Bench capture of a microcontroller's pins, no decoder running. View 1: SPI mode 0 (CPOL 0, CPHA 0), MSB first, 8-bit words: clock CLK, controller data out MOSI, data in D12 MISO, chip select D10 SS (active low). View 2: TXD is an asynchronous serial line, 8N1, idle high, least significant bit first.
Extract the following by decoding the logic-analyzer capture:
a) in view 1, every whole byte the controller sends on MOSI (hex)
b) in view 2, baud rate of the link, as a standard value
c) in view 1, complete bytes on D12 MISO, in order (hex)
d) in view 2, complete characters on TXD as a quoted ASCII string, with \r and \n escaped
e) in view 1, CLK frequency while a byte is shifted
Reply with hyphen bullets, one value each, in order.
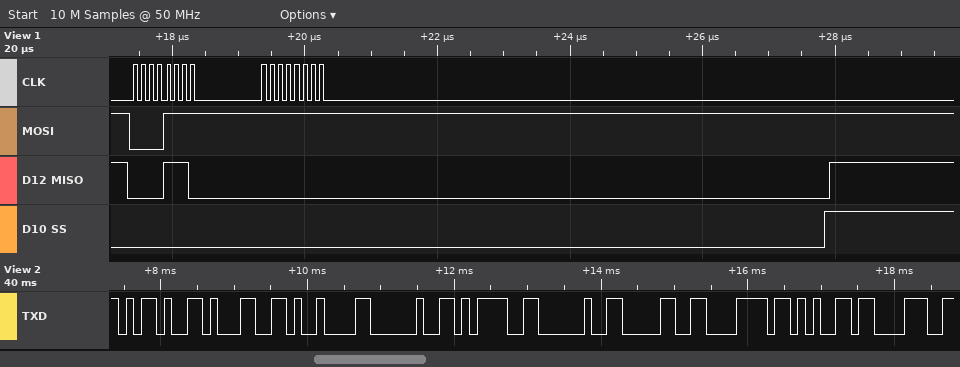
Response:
- 0F FF
- 9600 baud
- 0E 00
- "-1\t = 0xe8"
- 8 MHz
